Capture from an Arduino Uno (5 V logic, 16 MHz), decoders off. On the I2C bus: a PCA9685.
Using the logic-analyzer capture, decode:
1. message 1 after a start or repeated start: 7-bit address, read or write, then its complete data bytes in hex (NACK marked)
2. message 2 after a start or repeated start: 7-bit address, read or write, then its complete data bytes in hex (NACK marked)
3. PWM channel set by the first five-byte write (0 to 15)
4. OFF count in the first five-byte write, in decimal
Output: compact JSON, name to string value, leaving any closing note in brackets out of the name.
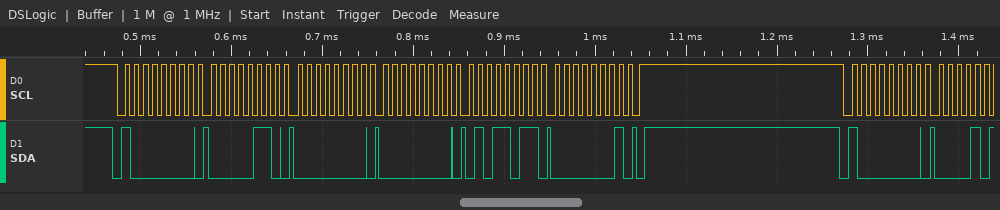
{"message 1 after a start or repeated start: 7-bit address, read or write, then its complete data bytes in hex": "0x40 write: 06 00 00 5B 01", "message 2 after a start or repeated start: 7-bit address, read or write, then its complete data bytes in hex": "0x40 write", "PWM channel set by the first five-byte write": "0", "OFF count in the first five-byte write, in decimal": "347"}
